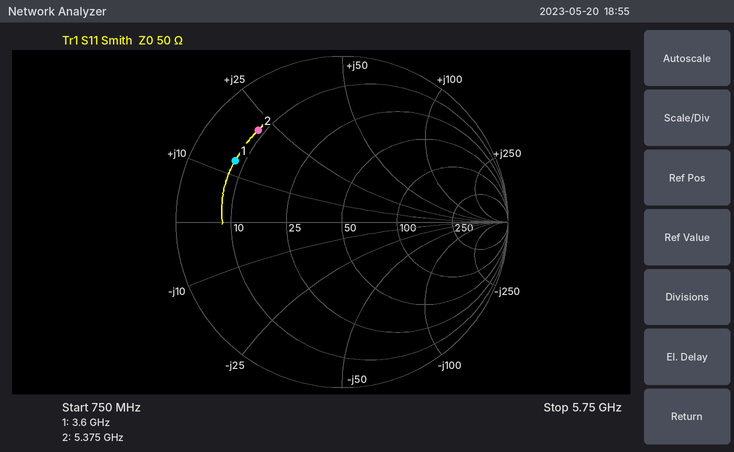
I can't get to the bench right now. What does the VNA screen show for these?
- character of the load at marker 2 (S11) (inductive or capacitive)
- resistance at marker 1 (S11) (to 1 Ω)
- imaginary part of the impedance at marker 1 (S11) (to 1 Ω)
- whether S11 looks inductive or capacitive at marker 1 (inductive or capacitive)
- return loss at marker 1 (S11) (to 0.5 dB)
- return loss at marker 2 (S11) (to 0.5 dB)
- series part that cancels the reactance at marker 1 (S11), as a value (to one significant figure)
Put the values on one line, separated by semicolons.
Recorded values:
inductive; 8 Ω; +13 Ω; inductive; 2.5 dB; 2.5 dB; 3 pF
